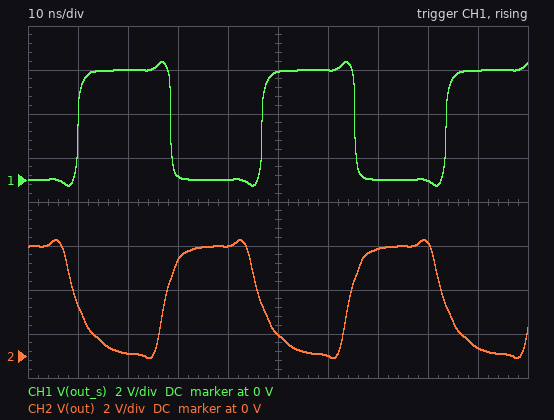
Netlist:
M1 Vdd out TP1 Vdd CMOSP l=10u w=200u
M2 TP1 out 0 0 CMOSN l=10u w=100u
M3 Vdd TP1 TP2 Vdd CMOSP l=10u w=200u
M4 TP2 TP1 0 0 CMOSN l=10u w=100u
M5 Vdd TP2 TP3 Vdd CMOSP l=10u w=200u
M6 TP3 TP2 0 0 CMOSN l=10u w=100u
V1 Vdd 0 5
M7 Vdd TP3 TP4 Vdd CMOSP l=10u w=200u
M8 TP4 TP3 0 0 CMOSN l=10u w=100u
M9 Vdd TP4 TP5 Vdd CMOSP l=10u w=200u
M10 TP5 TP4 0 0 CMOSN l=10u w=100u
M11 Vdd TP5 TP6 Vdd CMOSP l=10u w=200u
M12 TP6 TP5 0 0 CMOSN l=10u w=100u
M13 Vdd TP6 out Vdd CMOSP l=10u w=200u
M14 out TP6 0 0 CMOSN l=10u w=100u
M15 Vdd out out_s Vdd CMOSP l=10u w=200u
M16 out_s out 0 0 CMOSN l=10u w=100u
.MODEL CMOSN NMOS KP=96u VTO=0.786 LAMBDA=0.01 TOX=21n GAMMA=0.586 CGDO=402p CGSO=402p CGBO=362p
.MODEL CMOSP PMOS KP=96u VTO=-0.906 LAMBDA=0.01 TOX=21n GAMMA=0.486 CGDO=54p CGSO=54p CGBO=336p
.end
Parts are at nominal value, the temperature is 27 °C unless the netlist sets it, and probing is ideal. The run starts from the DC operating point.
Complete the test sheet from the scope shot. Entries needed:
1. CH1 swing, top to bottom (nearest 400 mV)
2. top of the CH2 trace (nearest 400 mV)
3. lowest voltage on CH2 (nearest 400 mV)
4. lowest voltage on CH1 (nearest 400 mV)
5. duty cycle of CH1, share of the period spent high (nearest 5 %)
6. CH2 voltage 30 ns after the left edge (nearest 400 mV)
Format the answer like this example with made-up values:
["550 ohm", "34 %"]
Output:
["5.6 V", "5.2 V", "0 V", "-400 mV", "50 %", "4.4 V"]
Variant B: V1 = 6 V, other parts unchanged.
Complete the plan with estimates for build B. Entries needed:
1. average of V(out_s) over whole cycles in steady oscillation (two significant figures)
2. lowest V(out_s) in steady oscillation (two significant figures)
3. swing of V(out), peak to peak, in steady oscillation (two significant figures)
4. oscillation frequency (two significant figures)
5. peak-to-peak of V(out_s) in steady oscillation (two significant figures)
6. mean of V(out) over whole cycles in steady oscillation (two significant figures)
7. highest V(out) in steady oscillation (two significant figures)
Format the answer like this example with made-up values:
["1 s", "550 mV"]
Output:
["3.0 V", "-300 mV", "6.4 V", "35 MHz", "6.7 V", "3.2 V", "6.3 V"]
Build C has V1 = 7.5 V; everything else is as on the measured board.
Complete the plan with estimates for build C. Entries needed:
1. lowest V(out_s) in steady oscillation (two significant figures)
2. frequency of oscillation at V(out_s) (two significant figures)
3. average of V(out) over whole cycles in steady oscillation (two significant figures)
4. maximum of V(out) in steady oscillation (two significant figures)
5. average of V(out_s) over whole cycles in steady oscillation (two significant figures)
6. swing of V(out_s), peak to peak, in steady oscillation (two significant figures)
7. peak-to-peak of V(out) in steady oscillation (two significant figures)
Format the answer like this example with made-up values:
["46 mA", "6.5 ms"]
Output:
["-370 mV", "47 MHz", "4.0 V", "7.9 V", "3.8 V", "8.4 V", "8.0 V"]
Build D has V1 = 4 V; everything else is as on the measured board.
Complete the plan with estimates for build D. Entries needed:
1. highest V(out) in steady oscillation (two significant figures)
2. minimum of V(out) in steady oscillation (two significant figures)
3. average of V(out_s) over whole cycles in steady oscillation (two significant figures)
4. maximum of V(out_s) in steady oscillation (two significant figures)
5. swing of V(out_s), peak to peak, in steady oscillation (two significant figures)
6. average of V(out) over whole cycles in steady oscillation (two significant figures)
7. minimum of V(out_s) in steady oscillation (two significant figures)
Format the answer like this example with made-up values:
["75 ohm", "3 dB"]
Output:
["4.2 V", "-98 mV", "2.0 V", "4.3 V", "4.5 V", "2.1 V", "-220 mV"]
